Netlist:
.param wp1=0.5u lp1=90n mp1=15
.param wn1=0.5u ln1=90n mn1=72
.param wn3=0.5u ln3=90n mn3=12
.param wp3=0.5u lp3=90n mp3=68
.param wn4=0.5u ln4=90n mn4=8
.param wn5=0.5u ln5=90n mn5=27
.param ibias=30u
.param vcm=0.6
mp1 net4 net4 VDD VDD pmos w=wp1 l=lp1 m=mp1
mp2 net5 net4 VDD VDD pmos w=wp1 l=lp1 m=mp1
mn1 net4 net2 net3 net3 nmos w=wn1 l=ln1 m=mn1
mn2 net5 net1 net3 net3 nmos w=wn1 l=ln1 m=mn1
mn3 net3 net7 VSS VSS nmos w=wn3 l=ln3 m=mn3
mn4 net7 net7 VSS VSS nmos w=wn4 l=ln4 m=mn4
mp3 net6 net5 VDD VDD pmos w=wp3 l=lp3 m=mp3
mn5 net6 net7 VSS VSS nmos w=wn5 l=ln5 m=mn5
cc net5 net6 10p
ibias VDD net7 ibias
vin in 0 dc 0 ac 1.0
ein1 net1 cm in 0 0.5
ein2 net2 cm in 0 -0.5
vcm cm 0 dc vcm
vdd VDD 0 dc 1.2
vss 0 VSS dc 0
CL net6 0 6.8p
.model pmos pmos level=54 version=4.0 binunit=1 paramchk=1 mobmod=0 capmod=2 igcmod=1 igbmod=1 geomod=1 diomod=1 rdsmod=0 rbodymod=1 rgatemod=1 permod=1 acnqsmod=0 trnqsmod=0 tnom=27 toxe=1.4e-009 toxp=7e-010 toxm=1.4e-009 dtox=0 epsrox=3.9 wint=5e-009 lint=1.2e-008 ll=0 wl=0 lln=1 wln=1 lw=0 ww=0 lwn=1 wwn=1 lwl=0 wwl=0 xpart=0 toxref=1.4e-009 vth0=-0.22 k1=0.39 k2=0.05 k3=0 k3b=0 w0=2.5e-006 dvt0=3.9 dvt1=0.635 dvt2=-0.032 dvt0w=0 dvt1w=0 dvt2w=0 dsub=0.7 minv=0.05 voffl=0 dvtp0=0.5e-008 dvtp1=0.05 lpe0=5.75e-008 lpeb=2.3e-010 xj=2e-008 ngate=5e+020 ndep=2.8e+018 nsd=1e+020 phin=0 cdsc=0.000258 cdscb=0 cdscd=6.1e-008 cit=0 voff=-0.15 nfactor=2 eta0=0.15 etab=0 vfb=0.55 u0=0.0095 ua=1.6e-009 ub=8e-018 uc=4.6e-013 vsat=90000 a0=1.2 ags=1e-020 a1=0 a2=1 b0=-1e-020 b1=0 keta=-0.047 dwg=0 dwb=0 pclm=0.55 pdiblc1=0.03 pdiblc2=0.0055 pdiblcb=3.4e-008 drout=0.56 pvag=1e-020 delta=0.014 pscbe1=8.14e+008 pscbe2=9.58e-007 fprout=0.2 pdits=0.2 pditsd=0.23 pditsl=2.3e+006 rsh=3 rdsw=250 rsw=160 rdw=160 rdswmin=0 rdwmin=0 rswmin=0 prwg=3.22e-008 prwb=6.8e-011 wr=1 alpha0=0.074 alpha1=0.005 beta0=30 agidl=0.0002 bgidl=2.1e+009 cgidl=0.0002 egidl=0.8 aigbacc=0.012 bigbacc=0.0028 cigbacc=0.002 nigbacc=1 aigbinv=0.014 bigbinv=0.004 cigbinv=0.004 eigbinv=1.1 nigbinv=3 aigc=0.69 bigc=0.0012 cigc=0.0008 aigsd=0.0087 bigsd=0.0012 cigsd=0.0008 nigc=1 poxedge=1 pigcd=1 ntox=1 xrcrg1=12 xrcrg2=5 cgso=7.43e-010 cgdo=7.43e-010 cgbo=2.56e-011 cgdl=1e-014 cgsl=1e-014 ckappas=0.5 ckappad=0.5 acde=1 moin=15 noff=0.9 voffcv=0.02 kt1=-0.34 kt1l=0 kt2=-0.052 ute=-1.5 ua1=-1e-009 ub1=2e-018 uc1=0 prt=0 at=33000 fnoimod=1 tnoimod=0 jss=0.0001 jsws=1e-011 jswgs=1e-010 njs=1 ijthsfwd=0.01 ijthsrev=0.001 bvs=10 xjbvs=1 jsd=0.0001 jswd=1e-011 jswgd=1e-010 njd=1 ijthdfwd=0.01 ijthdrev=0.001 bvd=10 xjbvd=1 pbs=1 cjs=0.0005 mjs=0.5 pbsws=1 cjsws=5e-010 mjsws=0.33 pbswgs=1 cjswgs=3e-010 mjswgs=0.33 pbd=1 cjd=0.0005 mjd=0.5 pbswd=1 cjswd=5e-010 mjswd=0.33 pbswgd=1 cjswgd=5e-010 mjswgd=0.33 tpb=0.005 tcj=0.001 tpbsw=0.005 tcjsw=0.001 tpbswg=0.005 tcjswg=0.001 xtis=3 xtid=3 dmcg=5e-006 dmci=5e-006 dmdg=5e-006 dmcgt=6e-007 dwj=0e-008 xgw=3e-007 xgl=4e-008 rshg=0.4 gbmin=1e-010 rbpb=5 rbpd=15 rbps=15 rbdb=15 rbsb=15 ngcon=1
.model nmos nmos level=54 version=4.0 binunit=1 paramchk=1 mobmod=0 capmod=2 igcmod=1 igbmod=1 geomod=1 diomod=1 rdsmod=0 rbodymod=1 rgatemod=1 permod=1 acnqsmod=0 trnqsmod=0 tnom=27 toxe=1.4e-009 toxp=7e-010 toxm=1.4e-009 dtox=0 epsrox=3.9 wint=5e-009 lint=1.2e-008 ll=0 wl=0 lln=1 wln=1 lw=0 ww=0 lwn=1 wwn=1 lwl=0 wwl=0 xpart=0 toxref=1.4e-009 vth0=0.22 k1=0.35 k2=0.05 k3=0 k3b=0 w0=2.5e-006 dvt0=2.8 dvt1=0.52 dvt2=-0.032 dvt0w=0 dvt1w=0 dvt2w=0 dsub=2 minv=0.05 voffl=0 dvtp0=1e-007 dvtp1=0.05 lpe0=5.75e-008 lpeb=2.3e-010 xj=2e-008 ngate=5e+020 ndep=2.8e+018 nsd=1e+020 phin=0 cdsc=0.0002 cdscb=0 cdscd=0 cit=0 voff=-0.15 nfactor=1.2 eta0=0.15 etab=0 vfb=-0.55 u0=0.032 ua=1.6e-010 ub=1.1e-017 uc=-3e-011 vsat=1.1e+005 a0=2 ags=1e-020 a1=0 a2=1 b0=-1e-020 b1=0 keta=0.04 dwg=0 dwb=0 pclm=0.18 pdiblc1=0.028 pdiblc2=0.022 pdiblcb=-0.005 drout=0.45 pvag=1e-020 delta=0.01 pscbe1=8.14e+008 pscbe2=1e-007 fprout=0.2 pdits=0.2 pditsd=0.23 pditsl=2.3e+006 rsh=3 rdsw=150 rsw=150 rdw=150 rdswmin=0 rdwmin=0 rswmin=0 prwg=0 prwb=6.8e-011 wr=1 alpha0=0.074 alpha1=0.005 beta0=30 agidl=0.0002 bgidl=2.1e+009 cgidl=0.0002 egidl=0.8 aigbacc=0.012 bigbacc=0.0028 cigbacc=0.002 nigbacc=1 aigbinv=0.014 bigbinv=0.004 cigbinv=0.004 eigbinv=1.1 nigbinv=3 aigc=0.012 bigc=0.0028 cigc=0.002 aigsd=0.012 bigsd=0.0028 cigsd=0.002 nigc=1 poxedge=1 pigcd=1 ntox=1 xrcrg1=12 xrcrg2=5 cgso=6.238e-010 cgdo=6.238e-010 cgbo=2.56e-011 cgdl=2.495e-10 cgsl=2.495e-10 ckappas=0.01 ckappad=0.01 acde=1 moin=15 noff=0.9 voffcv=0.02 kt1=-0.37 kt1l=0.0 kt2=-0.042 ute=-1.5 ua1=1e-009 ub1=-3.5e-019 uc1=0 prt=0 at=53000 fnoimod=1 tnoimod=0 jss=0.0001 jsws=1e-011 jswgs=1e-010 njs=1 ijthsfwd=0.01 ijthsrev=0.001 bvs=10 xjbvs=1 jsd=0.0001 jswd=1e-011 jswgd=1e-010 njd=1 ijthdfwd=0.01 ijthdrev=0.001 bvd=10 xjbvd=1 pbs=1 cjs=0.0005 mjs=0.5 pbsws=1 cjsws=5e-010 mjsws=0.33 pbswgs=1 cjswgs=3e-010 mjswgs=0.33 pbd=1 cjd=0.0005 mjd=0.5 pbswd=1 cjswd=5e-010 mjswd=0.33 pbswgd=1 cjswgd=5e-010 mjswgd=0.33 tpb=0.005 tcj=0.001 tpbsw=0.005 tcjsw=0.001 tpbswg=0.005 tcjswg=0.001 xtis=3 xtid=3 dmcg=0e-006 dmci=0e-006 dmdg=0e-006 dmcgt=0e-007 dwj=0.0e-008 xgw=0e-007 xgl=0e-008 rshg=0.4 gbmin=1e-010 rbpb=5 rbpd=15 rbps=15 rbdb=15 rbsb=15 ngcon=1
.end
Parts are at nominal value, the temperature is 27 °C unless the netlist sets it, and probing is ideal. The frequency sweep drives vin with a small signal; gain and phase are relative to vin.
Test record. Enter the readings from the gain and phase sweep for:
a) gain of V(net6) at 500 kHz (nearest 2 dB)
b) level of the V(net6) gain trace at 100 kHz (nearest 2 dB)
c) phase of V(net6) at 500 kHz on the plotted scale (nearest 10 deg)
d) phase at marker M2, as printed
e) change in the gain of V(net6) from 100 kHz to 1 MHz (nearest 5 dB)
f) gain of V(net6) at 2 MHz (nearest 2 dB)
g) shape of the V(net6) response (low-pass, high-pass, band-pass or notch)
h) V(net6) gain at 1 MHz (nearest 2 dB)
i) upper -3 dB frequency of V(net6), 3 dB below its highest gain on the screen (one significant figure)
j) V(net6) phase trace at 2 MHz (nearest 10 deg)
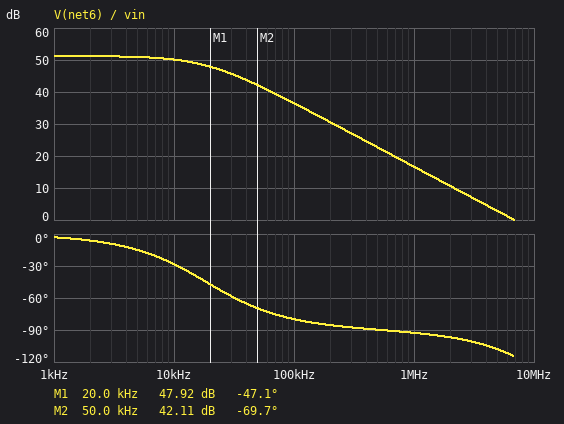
22 dB
36 dB
-90 deg
-69.7 deg
-20 dB
10 dB
low-pass
16 dB
20 kHz
-100 deg
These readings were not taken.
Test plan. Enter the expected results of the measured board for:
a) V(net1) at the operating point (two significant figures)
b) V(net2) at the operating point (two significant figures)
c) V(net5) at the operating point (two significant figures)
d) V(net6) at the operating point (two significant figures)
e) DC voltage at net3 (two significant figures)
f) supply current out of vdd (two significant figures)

600 mV
600 mV
820 mV
520 mV
340 mV
180 µA
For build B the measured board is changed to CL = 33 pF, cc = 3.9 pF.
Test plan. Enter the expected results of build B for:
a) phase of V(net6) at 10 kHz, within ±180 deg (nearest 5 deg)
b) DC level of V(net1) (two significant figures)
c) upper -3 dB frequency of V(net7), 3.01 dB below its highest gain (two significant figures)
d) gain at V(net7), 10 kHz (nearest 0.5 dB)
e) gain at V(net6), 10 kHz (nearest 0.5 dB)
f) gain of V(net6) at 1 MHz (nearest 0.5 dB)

-15 deg
600 mV
43 kHz
-24.0 dB
51.0 dB
24.0 dB
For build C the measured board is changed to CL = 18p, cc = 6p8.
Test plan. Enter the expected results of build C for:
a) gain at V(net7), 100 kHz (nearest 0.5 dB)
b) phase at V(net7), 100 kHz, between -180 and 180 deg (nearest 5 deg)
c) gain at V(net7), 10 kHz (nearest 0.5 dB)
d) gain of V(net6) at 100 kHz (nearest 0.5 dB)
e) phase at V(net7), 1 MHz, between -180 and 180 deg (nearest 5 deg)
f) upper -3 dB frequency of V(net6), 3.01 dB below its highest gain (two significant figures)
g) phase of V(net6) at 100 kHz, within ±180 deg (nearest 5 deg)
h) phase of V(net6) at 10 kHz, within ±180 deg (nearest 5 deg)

-35.5 dB
-70 deg
-24.5 dB
39.5 dB
-55 deg
27 kHz
-75 deg
-20 deg
